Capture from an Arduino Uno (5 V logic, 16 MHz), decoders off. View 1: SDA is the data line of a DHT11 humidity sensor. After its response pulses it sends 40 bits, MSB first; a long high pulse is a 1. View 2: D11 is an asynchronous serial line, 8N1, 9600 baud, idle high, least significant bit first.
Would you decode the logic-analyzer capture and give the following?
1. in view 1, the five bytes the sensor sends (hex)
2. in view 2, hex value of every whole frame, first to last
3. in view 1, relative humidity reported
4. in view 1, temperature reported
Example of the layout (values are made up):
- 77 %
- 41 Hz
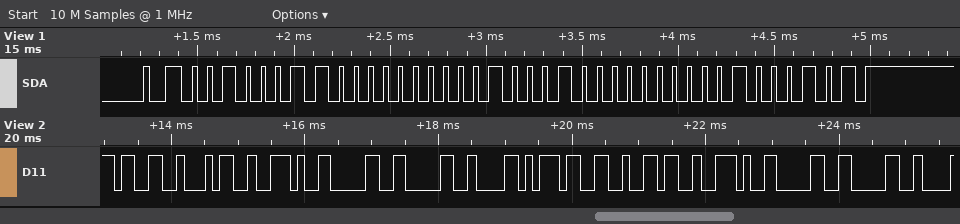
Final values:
- 23 00 22 00 45
- 0x33 0x34 0x2E 0x30 0x30 0x58 0x33 0x36 0x2E 0x30 0x30
- 35 %
- 34.0 °C
